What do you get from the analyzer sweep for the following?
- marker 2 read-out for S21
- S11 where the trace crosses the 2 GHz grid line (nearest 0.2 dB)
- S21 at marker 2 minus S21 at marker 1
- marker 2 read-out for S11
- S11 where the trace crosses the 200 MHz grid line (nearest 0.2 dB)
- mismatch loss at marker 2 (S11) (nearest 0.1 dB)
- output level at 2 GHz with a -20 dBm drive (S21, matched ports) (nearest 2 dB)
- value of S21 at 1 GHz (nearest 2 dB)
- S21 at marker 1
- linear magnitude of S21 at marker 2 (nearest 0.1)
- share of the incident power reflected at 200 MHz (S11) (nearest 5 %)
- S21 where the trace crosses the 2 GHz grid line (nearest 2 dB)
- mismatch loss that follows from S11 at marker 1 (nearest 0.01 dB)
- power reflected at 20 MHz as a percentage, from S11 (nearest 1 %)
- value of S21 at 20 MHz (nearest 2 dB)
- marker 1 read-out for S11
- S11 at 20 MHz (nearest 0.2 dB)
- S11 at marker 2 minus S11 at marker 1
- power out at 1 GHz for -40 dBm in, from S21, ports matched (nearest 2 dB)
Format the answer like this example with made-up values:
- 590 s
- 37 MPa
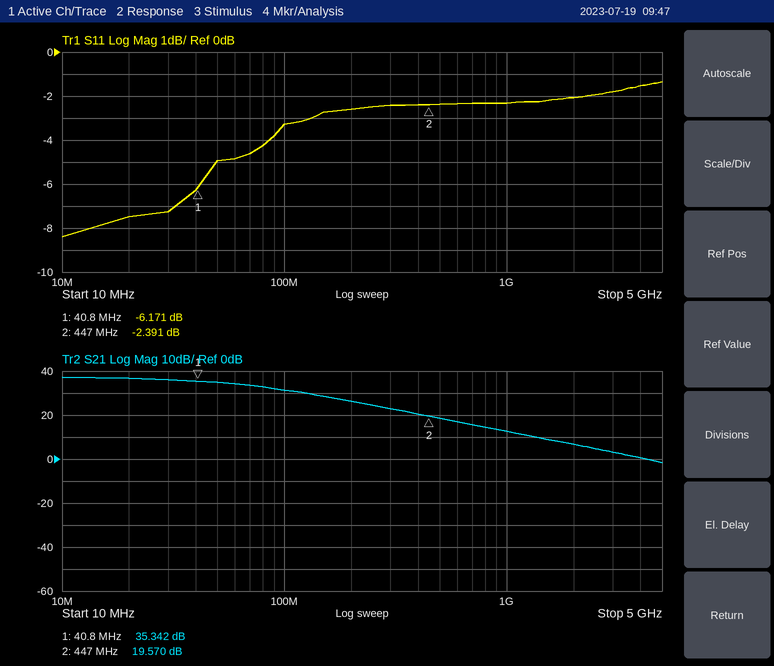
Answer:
- 19.570 dB
- -2.0 dB
- -15.772 dB
- -2.391 dB
- -2.6 dB
- 3.7 dB
- -14 dBm
- 12 dB
- 35.342 dB
- 9.5
- 55 %
- 6 dB
- 1.20 dB
- 18 %
- 36 dB
- -6.171 dB
- -7.4 dB
- 3.780 dB
- -28 dBm
